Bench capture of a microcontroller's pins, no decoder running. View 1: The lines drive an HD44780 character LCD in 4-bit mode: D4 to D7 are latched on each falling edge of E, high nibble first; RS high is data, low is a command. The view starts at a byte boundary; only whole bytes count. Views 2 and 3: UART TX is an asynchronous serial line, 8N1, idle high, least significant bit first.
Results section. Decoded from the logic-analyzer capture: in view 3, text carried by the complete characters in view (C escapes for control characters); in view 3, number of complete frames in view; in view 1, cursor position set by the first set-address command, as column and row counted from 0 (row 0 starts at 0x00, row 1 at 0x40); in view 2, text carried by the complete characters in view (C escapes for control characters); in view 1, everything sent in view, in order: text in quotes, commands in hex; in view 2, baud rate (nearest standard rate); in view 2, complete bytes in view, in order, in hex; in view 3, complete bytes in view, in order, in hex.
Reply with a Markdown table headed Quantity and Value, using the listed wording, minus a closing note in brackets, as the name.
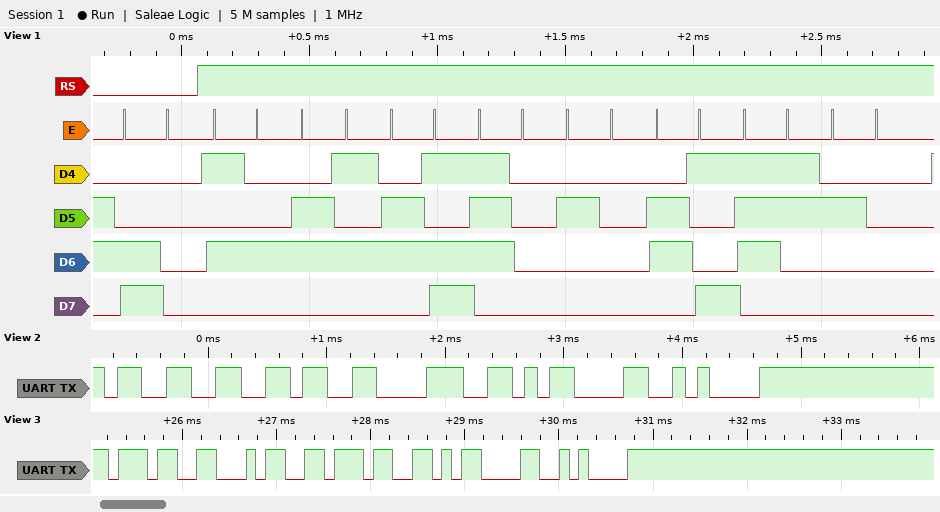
| Quantity | Value |
|---|---|
| in view 3, text carried by the complete characters in view | "747\r\n" |
| in view 3, number of complete frames in view | 5 |
| in view 1, cursor position set by the first set-address command, as column and row counted from 0 | column 0, row 1 |
| in view 2, text carried by the complete characters in view | "368\r\n" |
| in view 1, everything sent in view, in order: text in quotes, commands in hex | 0xC0 "Temp is " |
| in view 2, baud rate | 9600 baud |
| in view 2, complete bytes in view, in order, in hex | 33 36 38 0D 0A |
| in view 3, complete bytes in view, in order, in hex | 37 34 37 0D 0A |
